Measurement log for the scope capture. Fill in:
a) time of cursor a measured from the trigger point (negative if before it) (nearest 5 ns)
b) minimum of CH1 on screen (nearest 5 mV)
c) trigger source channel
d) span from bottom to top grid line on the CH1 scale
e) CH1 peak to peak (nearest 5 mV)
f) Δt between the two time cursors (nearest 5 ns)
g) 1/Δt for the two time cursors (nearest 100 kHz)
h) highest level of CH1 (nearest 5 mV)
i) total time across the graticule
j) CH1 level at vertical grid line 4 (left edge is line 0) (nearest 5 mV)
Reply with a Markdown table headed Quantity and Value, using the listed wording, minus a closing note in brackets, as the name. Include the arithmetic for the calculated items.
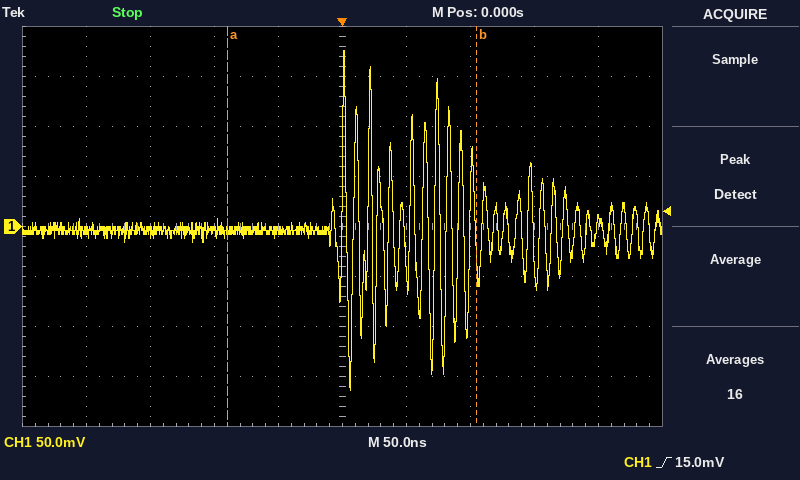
| Quantity | Value |
|---|---|
| time of cursor a measured from the trigger point (negative if before it) | -90 ns |
| minimum of CH1 on screen | -165 mV |
| trigger source channel | CH1 |
| span from bottom to top grid line on the CH1 scale | 400 mV |
| CH1 peak to peak | 175 mV − (-165 mV) = 340 mV |
| Δt between the two time cursors | 195 ns |
| 1/Δt for the two time cursors | 1 / 195 ns ≈ 5.1 MHz |
| highest level of CH1 | 175 mV |
| total time across the graticule | 500 ns |
| CH1 level at vertical grid line 4 (left edge is line 0) | -5 mV |
